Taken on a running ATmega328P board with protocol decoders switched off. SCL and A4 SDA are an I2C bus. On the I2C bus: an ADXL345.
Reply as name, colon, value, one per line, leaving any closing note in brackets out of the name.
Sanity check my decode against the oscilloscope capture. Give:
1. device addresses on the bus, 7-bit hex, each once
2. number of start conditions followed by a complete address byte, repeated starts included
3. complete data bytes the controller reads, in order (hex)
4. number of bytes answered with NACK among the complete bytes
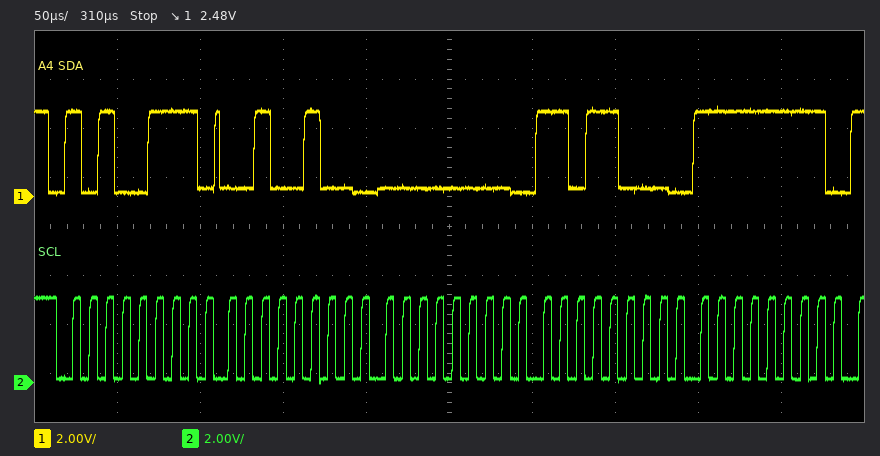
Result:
device addresses on the bus, 7-bit hex, each once: 0x53
number of start conditions followed by a complete address byte, repeated starts included: 1
complete data bytes the controller reads, in order: 24 00 D8 FF
number of bytes answered with NACK among the complete bytes: 0
